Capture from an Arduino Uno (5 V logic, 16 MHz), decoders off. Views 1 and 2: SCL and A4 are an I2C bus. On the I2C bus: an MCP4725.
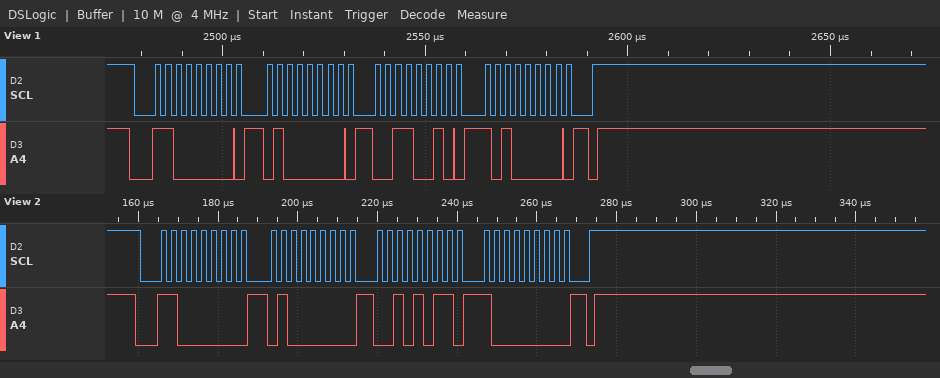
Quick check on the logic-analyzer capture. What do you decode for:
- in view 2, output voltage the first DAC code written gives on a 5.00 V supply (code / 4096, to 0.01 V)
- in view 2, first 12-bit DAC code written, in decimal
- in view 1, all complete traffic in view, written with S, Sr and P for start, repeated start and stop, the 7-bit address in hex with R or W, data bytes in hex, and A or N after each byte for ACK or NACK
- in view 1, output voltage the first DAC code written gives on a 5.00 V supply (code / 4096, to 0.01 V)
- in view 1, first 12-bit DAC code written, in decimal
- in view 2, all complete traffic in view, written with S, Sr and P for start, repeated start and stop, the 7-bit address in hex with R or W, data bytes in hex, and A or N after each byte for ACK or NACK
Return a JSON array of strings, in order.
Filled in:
["0.85 V", "696", "S 60W A 40 A 32 A A0 A P", "0.99 V", "810", "S 60W A 40 A 2B A 80 A P"]
